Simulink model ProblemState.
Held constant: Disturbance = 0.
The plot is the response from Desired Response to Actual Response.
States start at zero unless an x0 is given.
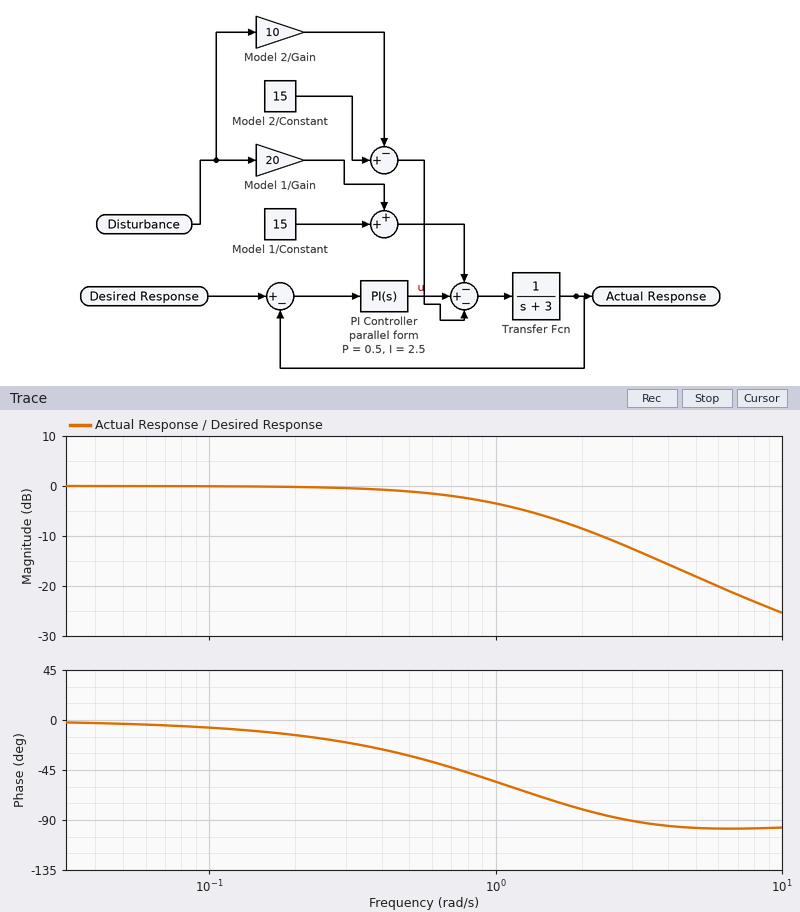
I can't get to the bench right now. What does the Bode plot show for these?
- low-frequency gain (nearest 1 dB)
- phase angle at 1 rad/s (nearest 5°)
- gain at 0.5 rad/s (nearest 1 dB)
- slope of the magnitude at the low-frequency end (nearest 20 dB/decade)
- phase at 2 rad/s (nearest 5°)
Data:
0 dB
-55°
-1 dB
0 dB/decade
-80°
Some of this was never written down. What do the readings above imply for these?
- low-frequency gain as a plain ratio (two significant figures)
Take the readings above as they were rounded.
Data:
1.0
